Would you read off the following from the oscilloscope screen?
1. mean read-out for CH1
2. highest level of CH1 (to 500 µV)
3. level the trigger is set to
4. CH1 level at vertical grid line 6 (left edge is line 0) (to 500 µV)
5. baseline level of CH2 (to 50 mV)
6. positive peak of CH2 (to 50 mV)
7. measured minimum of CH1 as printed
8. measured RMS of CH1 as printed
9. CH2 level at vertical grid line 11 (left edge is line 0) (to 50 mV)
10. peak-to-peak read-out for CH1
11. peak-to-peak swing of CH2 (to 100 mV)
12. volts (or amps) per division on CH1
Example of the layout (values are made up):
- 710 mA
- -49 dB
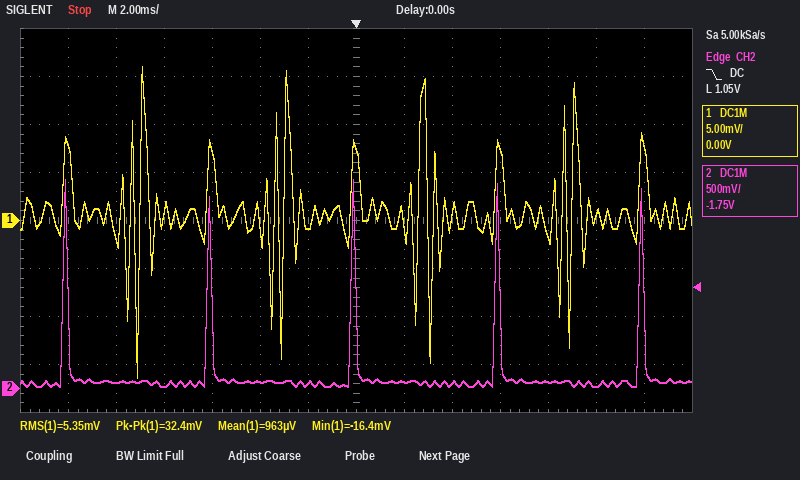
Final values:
- 963 µV
- 16.0 mV
- 1.05 V
- -1.0 mV
- 50 mV
- 2.20 V
- -16.4 mV
- 5.35 mV
- 50 mV
- 32.4 mV
- 2.20 V
- 5 mV
